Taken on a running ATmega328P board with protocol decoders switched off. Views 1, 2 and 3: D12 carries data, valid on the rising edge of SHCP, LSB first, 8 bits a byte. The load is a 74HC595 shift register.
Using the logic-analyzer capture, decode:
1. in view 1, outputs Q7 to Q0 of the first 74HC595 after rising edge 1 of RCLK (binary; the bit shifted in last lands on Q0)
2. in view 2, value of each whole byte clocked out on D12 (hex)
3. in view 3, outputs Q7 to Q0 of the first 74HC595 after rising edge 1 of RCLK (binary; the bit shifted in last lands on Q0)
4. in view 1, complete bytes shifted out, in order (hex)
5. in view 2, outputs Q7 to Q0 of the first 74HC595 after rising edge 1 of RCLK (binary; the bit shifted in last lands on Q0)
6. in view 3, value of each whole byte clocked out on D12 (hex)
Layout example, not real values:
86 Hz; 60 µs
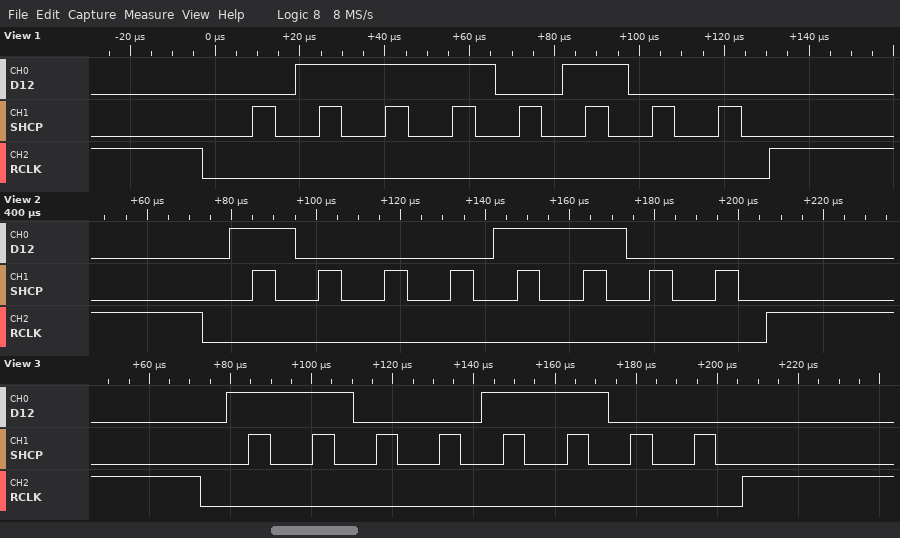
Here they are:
01110100; 31; 11001100; 2E; 10001100; 0x33
